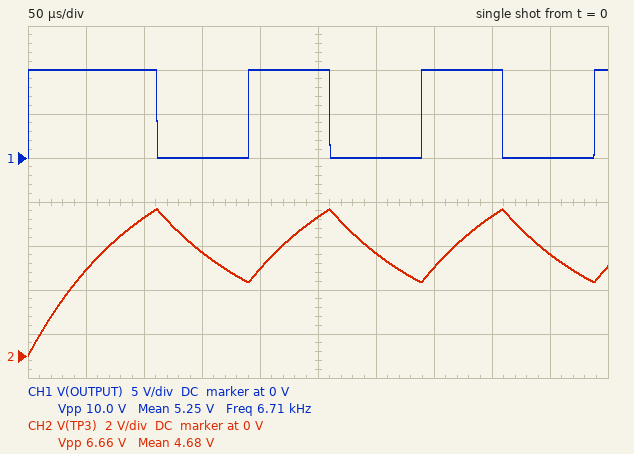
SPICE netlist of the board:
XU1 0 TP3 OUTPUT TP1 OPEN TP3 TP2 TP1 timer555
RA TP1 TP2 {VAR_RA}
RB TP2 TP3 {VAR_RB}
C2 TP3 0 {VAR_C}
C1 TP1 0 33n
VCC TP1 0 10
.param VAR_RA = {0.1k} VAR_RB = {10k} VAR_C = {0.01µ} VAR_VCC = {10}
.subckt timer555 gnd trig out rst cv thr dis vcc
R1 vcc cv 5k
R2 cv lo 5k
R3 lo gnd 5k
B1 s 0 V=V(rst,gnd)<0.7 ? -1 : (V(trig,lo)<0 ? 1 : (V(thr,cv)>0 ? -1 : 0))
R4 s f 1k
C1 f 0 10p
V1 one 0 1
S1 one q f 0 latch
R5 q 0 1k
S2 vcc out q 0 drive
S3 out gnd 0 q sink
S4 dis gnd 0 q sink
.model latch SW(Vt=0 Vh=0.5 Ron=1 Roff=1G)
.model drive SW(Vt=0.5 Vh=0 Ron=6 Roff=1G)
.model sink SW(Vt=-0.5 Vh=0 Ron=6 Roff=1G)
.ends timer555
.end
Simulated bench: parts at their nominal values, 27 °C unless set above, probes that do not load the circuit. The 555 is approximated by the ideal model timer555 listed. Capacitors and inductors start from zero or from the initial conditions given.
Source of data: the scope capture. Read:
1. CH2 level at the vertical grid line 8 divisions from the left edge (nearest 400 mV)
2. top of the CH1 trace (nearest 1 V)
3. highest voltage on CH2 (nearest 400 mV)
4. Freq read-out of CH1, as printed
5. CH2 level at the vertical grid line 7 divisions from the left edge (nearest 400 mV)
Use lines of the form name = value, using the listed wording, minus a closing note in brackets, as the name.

CH2 level at the vertical grid line 8 divisions from the left edge = 6.4 V
top of the CH1 trace = 10 V
highest voltage on CH2 = 6.8 V
Freq read-out of CH1, as printed = 6.71 kHz
CH2 level at the vertical grid line 7 divisions from the left edge = 4.0 V
